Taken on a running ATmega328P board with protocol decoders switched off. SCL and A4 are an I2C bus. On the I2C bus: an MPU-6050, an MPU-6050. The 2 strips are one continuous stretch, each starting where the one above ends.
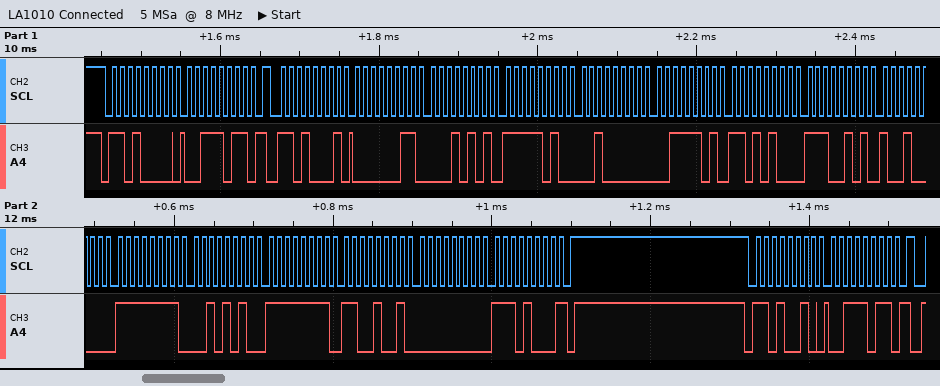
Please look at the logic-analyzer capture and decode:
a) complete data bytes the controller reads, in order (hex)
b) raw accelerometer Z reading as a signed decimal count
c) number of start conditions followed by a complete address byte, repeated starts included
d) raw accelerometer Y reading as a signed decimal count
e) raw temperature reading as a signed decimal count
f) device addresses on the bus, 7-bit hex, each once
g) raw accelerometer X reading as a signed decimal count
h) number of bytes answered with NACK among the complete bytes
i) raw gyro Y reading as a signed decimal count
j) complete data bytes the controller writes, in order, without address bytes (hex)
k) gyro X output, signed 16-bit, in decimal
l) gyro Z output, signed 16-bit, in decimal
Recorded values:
03 15 FA 20 3D D4 E5 90 FF 2A FF C9 00 E8
15828
3
-1504
-6768
0x68 0x69
789
1
-55
3B 3B
-214
232
